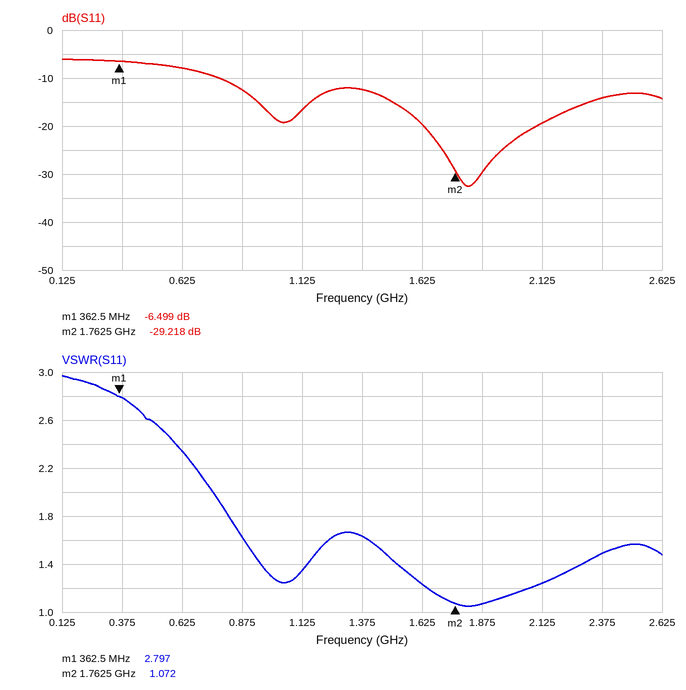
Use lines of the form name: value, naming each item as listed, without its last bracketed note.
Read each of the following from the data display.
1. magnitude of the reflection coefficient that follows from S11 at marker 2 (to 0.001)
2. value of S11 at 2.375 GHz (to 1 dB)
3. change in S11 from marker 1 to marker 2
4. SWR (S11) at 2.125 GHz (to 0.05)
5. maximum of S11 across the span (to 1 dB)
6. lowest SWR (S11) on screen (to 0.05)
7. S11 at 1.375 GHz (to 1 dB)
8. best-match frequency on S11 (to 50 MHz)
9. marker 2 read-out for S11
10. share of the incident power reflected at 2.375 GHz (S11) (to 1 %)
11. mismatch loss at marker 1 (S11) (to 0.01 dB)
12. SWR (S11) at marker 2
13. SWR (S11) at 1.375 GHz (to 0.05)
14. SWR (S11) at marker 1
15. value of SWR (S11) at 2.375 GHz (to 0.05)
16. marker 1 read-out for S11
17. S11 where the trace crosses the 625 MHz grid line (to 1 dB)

magnitude of the reflection coefficient that follows from S11 at marker 2: 0.035
value of S11 at 2.375 GHz: -14 dB
change in S11 from marker 1 to marker 2: -22.719 dB
SWR (S11) at 2.125 GHz: 1.25
maximum of S11 across the span: -6 dB
lowest SWR (S11) on screen: 1.05
S11 at 1.375 GHz: -12 dB
best-match frequency on S11: 1.80 GHz
marker 2 read-out for S11: -29.218 dB
share of the incident power reflected at 2.375 GHz (S11): 4 %
mismatch loss at marker 1 (S11): 1.10 dB
SWR (S11) at marker 2: 1.072
SWR (S11) at 1.375 GHz: 1.65
SWR (S11) at marker 1: 2.797
value of SWR (S11) at 2.375 GHz: 1.50
marker 1 read-out for S11: -6.499 dB
S11 where the trace crosses the 625 MHz grid line: -8 dB
